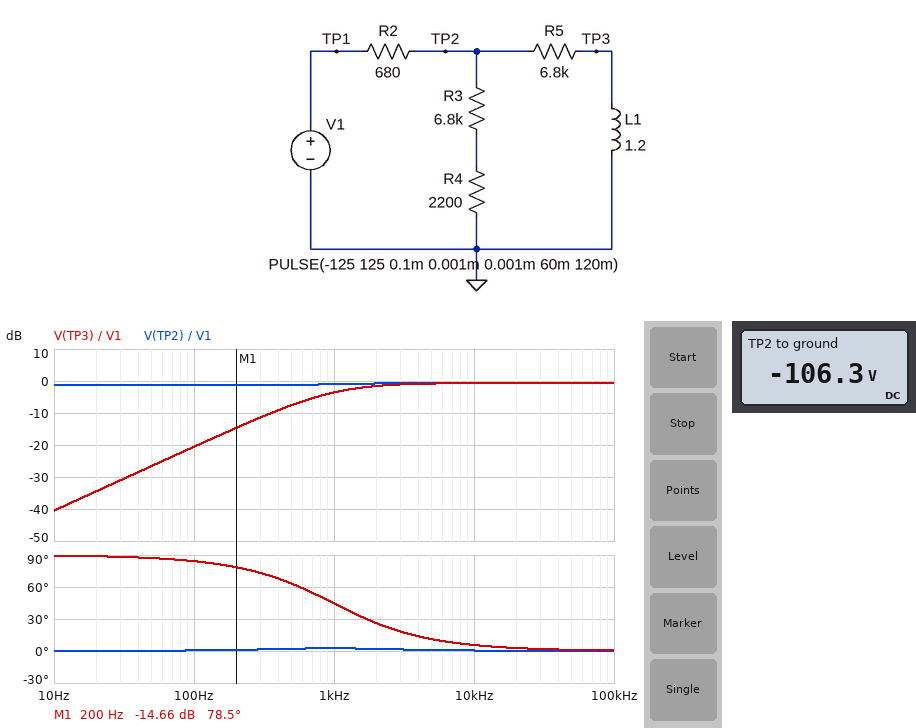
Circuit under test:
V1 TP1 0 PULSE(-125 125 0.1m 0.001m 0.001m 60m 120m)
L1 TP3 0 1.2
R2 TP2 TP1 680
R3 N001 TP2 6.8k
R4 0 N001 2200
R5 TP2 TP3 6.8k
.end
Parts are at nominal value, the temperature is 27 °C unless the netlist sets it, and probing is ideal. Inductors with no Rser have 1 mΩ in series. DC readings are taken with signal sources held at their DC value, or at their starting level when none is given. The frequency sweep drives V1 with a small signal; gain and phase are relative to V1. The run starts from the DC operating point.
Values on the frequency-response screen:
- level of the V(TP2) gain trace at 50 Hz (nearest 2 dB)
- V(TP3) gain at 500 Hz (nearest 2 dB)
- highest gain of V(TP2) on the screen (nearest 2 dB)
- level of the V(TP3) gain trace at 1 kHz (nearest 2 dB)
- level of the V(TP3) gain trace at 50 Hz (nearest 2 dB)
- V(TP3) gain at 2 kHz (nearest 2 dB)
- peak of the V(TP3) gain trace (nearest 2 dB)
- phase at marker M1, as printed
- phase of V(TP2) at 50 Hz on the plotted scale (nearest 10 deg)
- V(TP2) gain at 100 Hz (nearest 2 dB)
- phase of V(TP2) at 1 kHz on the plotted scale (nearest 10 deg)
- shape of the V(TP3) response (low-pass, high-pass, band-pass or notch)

-2 dB
-8 dB
0 dB
-4 dB
-26 dB
-2 dB
0 dB
78.5 deg
0 deg
-2 dB
0 deg
high-pass
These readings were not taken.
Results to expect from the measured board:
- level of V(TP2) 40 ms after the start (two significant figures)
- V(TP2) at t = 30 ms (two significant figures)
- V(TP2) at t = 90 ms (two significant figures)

110 V
110 V
-110 V
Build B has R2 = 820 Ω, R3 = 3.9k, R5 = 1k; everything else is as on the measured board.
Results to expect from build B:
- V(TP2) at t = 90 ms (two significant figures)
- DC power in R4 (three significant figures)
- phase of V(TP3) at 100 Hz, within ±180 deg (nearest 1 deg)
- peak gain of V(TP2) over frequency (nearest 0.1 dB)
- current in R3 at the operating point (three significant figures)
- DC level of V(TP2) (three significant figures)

-64 V
242 mW
66 deg
-1.1 dB
10.5 mA
-64.0 V
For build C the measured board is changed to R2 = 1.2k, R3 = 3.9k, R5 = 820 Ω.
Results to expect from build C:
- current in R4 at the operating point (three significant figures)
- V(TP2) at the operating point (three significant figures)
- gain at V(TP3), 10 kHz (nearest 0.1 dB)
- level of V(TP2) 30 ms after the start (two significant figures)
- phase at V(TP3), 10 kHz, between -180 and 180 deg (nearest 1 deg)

7.70 mA
-47.0 V
-1.6 dB
47 V
1 deg
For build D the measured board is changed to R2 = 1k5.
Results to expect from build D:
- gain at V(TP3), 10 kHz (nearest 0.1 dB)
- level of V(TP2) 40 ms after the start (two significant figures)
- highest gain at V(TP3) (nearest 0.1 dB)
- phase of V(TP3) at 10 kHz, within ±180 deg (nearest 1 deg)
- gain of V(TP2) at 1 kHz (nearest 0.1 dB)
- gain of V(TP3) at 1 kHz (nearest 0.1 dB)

-1.4 dB
90 V
-1.3 dB
6 deg
-2.1 dB
-4.7 dB
